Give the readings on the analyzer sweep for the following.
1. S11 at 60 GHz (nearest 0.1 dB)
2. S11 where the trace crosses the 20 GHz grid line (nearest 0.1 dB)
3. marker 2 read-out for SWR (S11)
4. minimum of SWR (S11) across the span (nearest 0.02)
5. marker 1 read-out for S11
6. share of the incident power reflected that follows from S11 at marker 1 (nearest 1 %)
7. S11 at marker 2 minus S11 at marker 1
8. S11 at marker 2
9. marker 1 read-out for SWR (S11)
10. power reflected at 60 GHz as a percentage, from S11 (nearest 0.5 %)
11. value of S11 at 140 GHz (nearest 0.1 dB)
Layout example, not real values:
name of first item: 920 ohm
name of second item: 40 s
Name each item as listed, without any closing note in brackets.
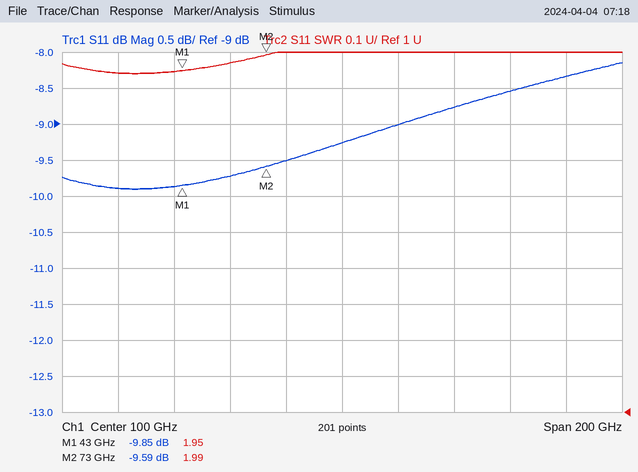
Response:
S11 at 60 GHz: -9.7 dB
S11 where the trace crosses the 20 GHz grid line: -9.9 dB
marker 2 read-out for SWR: 1.99
minimum of SWR (S11) across the span: 1.94
marker 1 read-out for S11: -9.85 dB
share of the incident power reflected that follows from S11 at marker 1: 10 %
S11 at marker 2 minus S11 at marker 1: 0.26 dB
S11 at marker 2: -9.59 dB
marker 1 read-out for SWR: 1.95
power reflected at 60 GHz as a percentage, from S11: 10.5 %
value of S11 at 140 GHz: -8.8 dB
